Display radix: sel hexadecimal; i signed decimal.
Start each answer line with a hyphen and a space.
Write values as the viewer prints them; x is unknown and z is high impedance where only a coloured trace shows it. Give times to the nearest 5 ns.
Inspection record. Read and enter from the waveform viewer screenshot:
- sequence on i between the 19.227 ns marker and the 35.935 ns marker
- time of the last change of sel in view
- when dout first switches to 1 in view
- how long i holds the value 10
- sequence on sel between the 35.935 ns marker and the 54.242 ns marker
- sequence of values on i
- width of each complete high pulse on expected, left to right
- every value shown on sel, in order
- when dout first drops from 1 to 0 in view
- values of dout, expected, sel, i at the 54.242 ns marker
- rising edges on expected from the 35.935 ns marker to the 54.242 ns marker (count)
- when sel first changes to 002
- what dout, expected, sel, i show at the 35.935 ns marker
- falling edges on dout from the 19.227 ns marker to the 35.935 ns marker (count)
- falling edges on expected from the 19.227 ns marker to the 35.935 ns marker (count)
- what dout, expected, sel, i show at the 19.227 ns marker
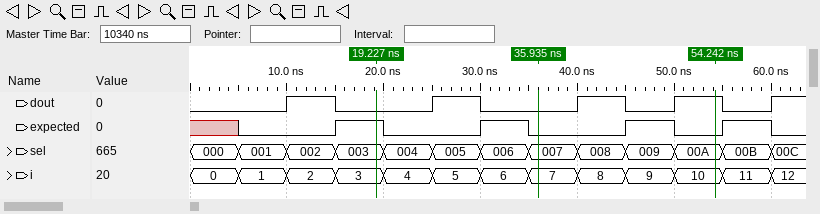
- 3, 4, 5, 6, 7
- 60 ns
- 10 ns
- 5 ns
- 007, 008, 009, 00A
- 0, 1, 2, 3, 4, 5, 6, 7, 8, 9, 10, 11, 12
- 5 ns, 5 ns, 5 ns, 5 ns
- 000, 001, 002, 003, 004, 005, 006, 007, 008, 009, 00A, 00B, 00C
- 15 ns
- dout=1, expected=0, sel=00A, i=10
- 1
- 10 ns
- dout=0, expected=0, sel=007, i=7
- 1
- 2
- dout=0, expected=1, sel=003, i=3
